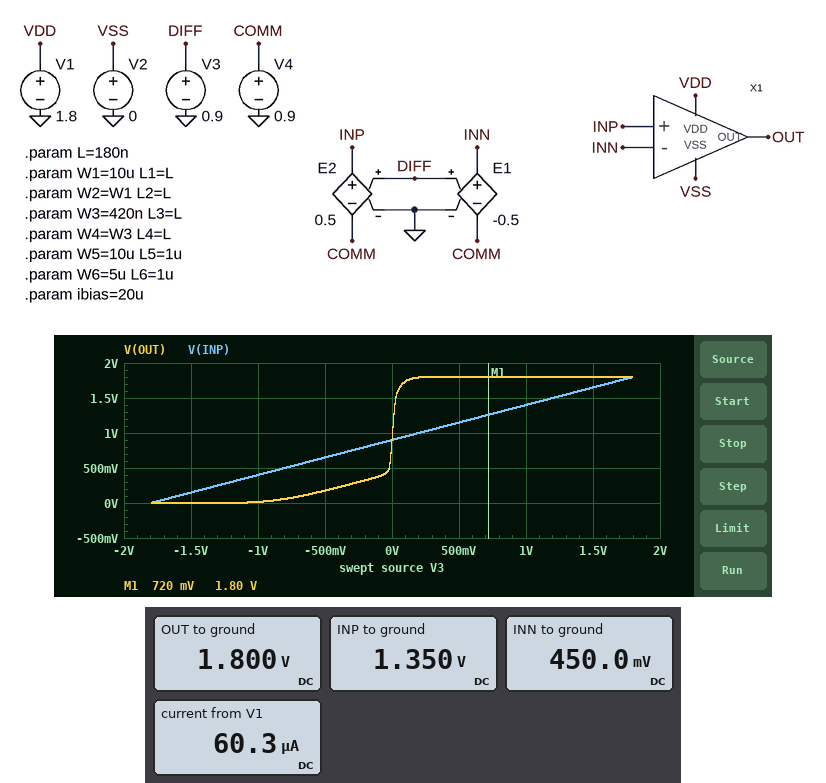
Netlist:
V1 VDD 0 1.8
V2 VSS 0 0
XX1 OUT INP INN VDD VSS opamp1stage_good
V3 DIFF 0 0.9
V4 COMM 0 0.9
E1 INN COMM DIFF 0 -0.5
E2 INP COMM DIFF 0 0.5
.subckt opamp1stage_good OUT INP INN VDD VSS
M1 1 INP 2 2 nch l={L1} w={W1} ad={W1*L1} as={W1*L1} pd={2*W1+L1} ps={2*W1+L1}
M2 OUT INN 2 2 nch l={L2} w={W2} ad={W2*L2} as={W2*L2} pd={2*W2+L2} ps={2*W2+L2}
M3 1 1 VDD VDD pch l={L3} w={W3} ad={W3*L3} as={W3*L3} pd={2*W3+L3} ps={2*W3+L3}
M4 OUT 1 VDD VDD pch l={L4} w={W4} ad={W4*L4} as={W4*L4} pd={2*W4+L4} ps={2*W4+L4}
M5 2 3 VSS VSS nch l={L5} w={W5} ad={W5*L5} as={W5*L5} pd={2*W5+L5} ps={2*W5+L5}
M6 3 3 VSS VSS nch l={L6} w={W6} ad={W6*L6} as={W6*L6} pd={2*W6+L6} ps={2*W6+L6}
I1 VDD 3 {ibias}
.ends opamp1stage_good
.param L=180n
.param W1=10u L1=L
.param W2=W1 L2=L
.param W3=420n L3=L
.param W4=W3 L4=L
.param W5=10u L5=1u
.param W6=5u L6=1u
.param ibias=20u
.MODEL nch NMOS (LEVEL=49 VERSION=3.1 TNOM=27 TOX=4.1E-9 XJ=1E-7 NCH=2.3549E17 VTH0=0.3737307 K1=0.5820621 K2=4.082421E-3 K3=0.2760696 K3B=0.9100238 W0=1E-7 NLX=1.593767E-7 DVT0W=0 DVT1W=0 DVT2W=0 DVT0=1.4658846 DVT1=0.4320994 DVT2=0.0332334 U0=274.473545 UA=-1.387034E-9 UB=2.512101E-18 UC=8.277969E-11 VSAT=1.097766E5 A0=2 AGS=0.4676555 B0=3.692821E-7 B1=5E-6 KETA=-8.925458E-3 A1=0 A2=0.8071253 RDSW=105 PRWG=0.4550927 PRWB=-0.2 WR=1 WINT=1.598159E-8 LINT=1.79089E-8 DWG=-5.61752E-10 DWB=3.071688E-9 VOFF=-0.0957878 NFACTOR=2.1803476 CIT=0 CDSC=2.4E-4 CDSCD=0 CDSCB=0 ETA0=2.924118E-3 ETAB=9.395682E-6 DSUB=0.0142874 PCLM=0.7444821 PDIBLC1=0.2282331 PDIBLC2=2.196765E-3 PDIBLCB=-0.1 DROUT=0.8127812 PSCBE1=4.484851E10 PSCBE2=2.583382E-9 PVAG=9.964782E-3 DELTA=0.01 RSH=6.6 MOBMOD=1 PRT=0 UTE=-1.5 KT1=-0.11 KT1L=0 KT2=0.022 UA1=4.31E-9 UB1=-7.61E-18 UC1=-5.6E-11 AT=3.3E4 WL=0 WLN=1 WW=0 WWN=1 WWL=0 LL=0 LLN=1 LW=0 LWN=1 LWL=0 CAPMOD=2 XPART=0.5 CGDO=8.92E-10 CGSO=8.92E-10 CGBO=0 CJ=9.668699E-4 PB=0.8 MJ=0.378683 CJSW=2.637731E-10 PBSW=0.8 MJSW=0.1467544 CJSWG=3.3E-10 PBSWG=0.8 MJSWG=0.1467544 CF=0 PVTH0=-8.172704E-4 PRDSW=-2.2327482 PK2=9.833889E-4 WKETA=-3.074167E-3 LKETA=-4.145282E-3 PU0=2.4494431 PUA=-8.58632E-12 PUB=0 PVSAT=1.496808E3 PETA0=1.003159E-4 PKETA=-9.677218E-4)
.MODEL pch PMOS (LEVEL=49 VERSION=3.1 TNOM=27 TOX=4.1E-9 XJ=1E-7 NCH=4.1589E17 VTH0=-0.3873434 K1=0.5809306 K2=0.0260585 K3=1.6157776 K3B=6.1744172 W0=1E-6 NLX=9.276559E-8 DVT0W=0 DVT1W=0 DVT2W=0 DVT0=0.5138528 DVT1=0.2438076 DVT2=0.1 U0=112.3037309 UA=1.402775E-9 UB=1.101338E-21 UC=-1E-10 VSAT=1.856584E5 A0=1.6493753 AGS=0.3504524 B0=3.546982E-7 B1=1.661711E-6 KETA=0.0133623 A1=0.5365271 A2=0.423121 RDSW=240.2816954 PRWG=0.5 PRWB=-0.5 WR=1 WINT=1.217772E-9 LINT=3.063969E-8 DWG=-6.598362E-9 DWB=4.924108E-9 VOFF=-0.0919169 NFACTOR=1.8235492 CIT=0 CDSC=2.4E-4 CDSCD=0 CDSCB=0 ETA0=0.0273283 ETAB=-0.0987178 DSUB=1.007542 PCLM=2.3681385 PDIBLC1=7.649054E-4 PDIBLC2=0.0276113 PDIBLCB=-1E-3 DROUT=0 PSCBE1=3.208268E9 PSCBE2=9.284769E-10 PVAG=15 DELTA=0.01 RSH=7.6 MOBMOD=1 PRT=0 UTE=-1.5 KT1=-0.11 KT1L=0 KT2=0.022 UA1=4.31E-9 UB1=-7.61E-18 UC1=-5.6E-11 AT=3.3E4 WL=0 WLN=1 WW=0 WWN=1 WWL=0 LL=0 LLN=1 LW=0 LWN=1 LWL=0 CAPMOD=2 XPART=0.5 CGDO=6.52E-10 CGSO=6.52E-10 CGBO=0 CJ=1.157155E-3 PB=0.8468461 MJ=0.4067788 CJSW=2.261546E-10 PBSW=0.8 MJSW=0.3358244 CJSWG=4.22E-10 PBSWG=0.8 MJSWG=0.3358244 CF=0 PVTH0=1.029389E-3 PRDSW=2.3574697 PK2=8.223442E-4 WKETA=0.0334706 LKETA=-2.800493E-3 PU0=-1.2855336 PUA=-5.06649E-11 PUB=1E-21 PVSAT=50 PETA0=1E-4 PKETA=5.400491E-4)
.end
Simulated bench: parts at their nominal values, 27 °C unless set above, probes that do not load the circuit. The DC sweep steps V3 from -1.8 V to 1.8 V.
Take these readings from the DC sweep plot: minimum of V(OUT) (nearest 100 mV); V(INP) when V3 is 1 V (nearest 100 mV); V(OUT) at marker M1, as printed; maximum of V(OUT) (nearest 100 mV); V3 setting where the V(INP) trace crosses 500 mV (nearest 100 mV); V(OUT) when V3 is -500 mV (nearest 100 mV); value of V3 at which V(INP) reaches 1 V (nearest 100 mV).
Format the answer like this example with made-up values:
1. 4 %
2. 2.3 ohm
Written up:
1. 0 V
2. 1.4 V
3. 1.80 V
4. 1.8 V
5. -800 mV
6. 200 mV
7. 200 mV
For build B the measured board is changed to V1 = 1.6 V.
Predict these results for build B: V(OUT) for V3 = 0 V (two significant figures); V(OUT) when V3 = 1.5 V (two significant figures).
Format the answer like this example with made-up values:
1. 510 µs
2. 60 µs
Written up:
1. 700 mV
2. 1.6 V
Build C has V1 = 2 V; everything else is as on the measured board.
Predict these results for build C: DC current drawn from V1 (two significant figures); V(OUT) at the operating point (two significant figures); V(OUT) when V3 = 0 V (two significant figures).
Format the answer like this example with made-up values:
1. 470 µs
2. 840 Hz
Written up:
1. 61 µA
2. 2.0 V
3. 1.1 V
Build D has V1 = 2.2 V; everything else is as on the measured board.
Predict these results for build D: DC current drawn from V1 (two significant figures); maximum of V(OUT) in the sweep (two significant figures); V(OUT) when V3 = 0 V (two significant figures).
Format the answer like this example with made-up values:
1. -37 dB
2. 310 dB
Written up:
1. 61 µA
2. 2.2 V
3. 1.3 V
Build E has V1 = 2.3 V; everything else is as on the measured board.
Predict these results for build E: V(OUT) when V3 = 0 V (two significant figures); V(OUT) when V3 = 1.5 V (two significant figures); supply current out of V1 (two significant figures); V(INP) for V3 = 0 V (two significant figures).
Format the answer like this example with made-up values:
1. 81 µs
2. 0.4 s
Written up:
1. 1.4 V
2. 2.3 V
3. 61 µA
4. 900 mV
